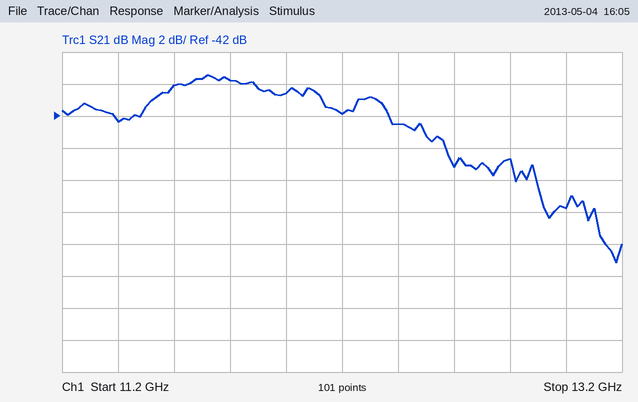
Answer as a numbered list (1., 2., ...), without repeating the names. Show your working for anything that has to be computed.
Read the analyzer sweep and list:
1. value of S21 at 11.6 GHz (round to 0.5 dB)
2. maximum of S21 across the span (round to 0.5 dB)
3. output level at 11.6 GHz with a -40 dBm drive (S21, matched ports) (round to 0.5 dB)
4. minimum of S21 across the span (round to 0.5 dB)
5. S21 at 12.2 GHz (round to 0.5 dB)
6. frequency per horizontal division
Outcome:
1. -40.0 dB
2. -39.5 dB
3. -40 dBm + (-40.0 dB) = -80.0 dBm
4. -51.0 dB
5. -42.0 dB
6. 200 MHz
